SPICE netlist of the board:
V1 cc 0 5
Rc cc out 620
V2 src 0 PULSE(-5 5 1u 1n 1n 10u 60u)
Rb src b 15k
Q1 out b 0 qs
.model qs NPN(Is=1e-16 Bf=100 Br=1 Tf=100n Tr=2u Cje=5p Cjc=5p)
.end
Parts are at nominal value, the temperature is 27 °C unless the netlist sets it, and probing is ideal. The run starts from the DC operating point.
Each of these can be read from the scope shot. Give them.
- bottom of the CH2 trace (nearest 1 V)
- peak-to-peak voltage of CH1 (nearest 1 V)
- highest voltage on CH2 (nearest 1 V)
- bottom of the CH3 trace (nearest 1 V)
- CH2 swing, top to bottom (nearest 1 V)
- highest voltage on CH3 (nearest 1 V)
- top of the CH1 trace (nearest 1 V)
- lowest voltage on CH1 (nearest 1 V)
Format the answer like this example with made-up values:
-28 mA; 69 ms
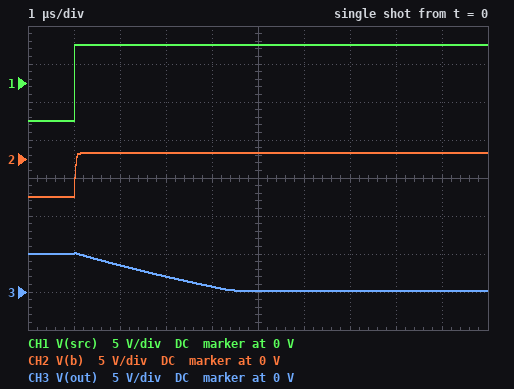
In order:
-5 V; 10 V; 1 V; 0 V; 6 V; 5 V; 5 V; -5 V
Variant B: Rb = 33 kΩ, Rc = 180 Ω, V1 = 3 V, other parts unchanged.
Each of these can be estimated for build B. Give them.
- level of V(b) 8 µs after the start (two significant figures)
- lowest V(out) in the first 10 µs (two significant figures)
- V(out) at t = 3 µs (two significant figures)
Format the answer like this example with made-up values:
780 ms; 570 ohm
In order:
820 mV; 1.7 V; 2.6 V
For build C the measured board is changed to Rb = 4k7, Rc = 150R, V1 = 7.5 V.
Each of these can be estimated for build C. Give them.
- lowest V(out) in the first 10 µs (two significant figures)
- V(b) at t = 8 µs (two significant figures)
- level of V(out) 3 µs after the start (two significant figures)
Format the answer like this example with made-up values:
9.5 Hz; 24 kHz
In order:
160 mV; 870 mV; 5.1 V
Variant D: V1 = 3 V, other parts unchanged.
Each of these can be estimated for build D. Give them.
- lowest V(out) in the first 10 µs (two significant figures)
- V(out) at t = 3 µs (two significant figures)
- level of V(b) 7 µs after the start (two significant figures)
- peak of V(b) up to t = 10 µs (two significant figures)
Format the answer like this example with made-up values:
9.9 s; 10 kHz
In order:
82 mV; 180 mV; 820 mV; 820 mV
